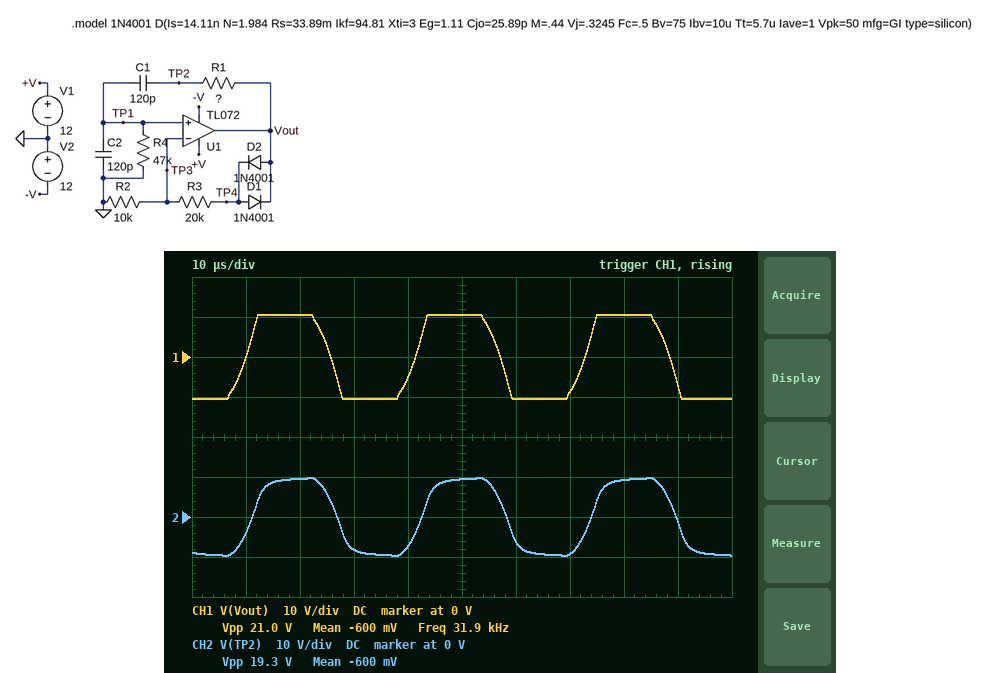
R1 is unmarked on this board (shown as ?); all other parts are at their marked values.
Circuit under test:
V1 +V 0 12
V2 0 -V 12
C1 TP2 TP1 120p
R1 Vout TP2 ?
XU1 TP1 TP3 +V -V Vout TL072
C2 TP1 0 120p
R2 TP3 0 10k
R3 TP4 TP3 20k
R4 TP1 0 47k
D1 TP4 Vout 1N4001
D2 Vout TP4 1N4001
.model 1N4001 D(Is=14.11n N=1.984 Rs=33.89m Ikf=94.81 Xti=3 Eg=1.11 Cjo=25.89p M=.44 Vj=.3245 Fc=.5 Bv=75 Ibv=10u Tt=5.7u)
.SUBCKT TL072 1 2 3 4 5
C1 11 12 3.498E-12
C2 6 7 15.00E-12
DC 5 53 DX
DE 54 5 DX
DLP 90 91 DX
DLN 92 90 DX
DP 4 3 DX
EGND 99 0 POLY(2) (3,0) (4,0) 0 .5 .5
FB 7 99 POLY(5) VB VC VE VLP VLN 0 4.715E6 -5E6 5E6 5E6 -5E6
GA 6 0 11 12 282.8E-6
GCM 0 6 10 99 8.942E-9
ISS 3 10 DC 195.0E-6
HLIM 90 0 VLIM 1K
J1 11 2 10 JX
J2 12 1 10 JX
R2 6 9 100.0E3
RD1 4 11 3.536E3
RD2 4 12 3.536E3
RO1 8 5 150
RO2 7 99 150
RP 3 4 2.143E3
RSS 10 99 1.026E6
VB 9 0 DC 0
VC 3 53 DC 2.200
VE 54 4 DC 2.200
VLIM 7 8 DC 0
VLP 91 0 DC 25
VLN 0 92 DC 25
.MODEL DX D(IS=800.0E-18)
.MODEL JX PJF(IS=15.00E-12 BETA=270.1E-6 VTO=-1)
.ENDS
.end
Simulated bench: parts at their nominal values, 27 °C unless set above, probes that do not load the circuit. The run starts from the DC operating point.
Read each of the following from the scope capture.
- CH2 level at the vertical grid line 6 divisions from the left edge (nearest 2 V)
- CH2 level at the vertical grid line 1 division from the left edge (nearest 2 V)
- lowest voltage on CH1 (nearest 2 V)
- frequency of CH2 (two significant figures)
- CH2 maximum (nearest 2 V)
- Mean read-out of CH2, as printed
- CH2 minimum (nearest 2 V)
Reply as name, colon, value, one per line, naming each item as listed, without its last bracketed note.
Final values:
CH2 level at the vertical grid line 6 divisions from the left edge: -6 V
CH2 level at the vertical grid line 1 division from the left edge: -4 V
lowest voltage on CH1: -10 V
frequency of CH2: 32 kHz
CH2 maximum: 10 V
Mean read-out of CH2, as printed: -600 mV
CH2 minimum: -10 V
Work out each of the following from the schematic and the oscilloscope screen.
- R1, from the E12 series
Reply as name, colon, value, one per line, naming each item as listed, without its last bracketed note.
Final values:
R1, from the E12 series: 22 kΩ
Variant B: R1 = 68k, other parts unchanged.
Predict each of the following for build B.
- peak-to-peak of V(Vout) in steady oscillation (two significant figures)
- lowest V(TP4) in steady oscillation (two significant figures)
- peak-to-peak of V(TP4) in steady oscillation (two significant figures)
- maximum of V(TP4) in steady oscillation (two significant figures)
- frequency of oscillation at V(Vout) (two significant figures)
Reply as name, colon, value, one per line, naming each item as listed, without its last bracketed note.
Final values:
peak-to-peak of V(Vout) in steady oscillation: 6.6 V
lowest V(TP4) in steady oscillation: -2.9 V
peak-to-peak of V(TP4) in steady oscillation: 5.7 V
maximum of V(TP4) in steady oscillation: 2.9 V
frequency of oscillation at V(Vout): 20 kHz
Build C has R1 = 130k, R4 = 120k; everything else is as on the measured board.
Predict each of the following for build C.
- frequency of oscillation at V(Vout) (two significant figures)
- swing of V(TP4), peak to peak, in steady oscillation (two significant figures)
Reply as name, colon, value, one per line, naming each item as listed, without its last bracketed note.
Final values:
frequency of oscillation at V(Vout): 10 kHz
swing of V(TP4), peak to peak, in steady oscillation: 20 V
